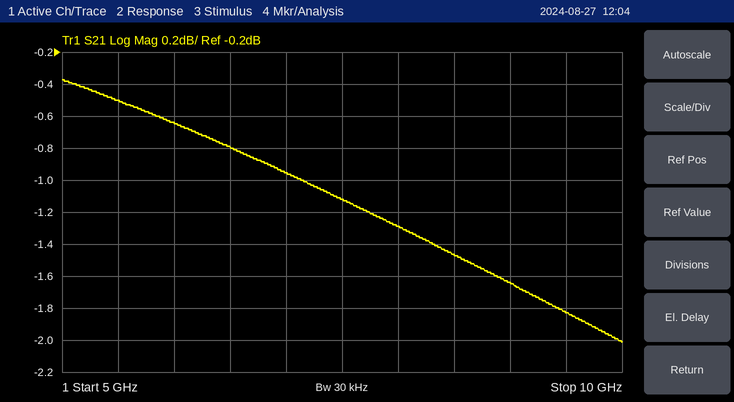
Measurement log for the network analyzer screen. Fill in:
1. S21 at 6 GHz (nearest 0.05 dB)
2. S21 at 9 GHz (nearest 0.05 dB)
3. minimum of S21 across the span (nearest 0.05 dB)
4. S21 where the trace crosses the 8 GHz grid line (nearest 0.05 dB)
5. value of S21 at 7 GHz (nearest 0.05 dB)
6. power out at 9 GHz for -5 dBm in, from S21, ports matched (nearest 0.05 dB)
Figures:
-0.65 dB
-1.65 dB
-2.00 dB
-1.30 dB
-0.95 dB
-6.65 dBm
